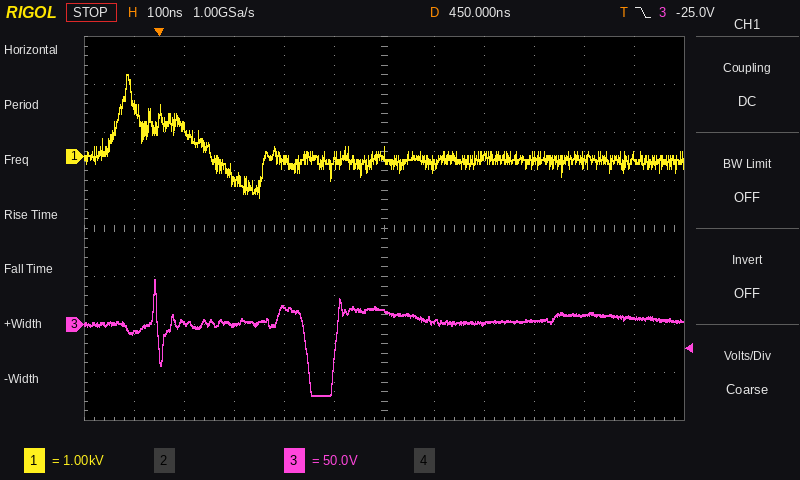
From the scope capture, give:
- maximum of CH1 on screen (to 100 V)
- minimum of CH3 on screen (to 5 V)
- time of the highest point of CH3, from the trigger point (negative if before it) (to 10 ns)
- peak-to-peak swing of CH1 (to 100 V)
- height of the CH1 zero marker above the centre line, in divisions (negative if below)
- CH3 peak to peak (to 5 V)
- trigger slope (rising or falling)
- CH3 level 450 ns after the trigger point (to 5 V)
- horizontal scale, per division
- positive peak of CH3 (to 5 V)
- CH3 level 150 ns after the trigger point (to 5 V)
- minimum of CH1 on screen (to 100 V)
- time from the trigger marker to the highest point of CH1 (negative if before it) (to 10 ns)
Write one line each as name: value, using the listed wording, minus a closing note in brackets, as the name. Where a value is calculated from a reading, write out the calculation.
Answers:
maximum of CH1 on screen: 1.7 kV
minimum of CH3 on screen: -75 V
time of the highest point of CH3, from the trigger point (negative if before it): -10 ns
peak-to-peak swing of CH1: 1.7 kV − (-900 V) = 2.6 kV
height of the CH1 zero marker above the centre line, in divisions: +1.5 div
CH3 peak to peak: 45 V − (-75 V) = 120 V
trigger slope: falling
CH3 level 450 ns after the trigger point: 15 V
horizontal scale, per division: 100 ns
positive peak of CH3: 45 V
CH3 level 150 ns after the trigger point: 0 V
minimum of CH1 on screen: -900 V
time from the trigger marker to the highest point of CH1 (negative if before it): -60 ns
